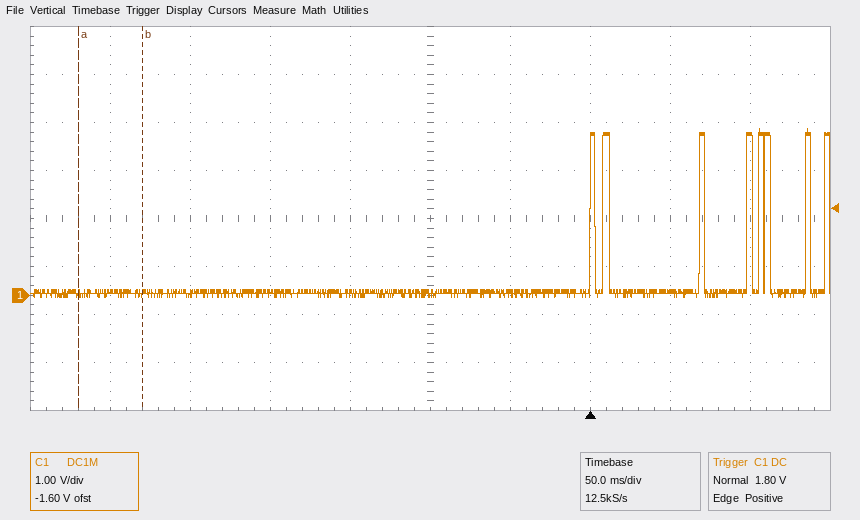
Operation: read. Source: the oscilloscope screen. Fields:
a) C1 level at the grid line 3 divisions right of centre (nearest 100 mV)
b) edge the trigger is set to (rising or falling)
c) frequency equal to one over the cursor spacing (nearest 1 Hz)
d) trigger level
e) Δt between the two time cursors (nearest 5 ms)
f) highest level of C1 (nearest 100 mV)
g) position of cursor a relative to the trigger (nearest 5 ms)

100 mV
rising
25 Hz
1.80 V
40 ms
3.5 V
-320 ms
